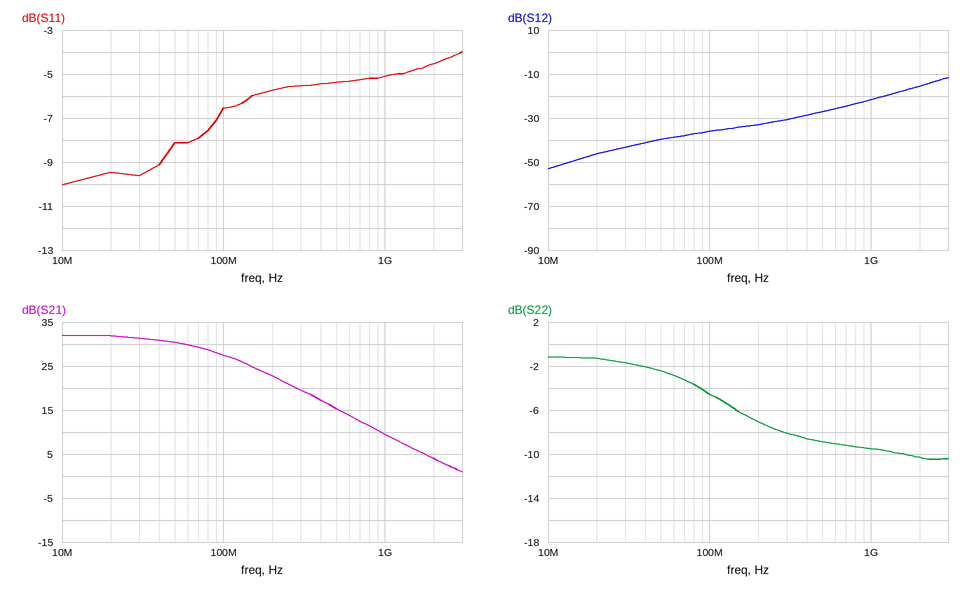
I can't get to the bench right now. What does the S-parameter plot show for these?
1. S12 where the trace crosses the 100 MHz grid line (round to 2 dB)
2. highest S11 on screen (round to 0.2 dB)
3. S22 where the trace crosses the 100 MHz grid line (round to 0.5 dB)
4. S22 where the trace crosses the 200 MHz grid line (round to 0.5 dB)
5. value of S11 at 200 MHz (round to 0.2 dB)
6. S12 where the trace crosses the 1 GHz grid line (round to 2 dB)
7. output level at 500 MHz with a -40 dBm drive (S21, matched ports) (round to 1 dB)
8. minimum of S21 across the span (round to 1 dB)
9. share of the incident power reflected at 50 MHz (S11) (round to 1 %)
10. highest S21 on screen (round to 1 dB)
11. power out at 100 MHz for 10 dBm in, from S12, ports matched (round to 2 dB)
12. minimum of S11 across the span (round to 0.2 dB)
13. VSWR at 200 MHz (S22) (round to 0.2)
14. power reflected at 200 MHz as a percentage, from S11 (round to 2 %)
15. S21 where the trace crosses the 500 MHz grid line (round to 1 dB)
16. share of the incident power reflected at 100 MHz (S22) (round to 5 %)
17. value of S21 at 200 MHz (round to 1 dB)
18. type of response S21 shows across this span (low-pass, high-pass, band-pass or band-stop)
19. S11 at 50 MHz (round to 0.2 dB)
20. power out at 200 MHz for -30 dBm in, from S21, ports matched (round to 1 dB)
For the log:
-36 dB
-4.0 dB
-4.5 dB
-7.0 dB
-5.8 dB
-22 dB
-25 dBm
1 dB
15 %
32 dB
-26 dBm
-10.0 dB
2.6
26 %
15 dB
35 %
23 dB
low-pass
-8.2 dB
-7 dBm
